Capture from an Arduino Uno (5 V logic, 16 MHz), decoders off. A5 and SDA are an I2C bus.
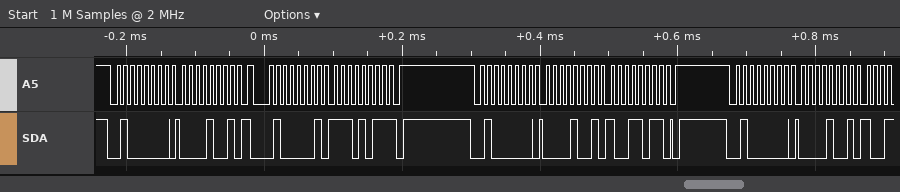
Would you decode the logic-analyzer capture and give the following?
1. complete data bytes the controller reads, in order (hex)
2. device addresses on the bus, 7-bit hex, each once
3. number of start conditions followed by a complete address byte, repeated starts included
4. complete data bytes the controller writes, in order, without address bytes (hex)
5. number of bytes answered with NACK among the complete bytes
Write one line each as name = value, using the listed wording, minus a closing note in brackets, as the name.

complete data bytes the controller reads, in order = EB
device addresses on the bus, 7-bit hex, each once = 0x20
number of start conditions followed by a complete address byte, repeated starts included = 4
complete data bytes the controller writes, in order, without address bytes = 09 09 9B 09
number of bytes answered with NACK among the complete bytes = 1
